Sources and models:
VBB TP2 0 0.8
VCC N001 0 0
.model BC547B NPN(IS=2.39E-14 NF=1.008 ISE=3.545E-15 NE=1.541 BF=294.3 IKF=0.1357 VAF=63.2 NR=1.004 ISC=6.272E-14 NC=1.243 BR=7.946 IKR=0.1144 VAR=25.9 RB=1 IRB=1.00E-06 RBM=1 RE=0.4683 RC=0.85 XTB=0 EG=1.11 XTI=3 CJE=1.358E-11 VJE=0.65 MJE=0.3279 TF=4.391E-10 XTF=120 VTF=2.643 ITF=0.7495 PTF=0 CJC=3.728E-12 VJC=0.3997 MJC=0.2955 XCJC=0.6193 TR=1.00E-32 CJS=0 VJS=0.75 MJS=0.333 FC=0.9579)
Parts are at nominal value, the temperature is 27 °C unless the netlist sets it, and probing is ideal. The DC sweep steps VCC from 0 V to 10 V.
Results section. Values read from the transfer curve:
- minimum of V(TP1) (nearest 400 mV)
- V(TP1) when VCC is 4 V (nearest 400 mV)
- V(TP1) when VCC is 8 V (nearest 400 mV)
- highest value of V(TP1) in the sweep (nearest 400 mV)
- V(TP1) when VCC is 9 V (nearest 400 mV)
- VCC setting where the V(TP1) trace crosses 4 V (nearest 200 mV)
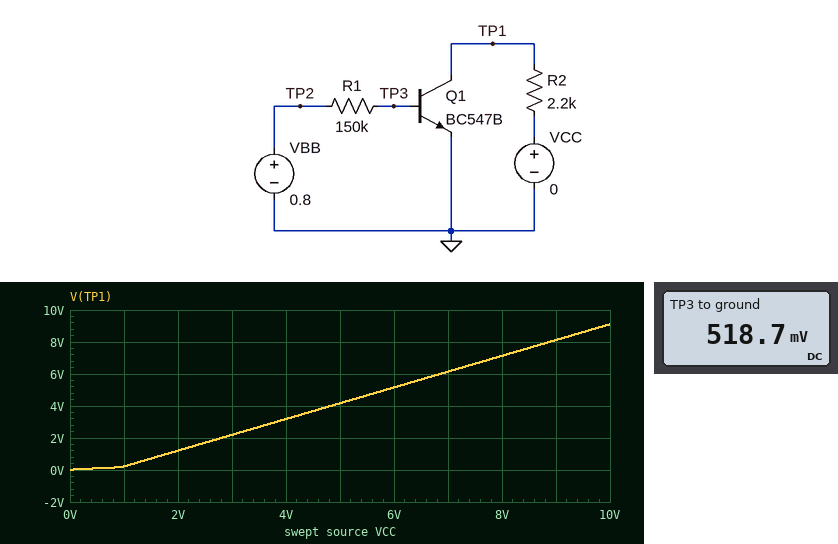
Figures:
0 V
3.2 V
7.2 V
9.2 V
8.0 V
4.8 V
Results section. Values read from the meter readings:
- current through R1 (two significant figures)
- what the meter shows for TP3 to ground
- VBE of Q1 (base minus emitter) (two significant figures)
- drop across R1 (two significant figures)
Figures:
1.9 µA
518.7 mV
520 mV
280 mV
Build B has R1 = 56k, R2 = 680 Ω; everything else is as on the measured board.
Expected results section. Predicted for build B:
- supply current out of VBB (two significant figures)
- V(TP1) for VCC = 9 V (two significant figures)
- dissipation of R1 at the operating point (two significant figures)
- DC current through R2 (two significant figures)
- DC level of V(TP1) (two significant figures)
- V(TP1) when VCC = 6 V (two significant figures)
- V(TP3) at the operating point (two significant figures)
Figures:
4.6 µA
8.4 V
1.2 µW
4.0 µA
2.7 mV
5.4 V
540 mV
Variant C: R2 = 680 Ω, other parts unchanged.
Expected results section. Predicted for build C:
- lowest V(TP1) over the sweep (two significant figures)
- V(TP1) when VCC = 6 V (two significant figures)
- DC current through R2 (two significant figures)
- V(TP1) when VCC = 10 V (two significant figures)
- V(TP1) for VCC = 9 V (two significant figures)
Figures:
1.4 mV
5.7 V
2.1 µA
9.7 V
8.7 V
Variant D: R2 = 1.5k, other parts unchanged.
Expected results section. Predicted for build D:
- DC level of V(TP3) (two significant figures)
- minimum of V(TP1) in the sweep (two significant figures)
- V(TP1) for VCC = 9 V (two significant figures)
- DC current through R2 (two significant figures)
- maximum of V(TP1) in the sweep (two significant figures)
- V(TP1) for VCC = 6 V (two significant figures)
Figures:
520 mV
2.5 mV
8.4 V
1.7 µA
9.4 V
5.4 V
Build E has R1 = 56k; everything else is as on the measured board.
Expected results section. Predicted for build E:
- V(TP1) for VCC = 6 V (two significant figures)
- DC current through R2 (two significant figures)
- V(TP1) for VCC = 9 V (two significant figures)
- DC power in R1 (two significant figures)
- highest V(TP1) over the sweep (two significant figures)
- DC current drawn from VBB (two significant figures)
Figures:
4.1 V
2.1 µA
7.0 V
1.2 µW
7.9 V
4.6 µA
